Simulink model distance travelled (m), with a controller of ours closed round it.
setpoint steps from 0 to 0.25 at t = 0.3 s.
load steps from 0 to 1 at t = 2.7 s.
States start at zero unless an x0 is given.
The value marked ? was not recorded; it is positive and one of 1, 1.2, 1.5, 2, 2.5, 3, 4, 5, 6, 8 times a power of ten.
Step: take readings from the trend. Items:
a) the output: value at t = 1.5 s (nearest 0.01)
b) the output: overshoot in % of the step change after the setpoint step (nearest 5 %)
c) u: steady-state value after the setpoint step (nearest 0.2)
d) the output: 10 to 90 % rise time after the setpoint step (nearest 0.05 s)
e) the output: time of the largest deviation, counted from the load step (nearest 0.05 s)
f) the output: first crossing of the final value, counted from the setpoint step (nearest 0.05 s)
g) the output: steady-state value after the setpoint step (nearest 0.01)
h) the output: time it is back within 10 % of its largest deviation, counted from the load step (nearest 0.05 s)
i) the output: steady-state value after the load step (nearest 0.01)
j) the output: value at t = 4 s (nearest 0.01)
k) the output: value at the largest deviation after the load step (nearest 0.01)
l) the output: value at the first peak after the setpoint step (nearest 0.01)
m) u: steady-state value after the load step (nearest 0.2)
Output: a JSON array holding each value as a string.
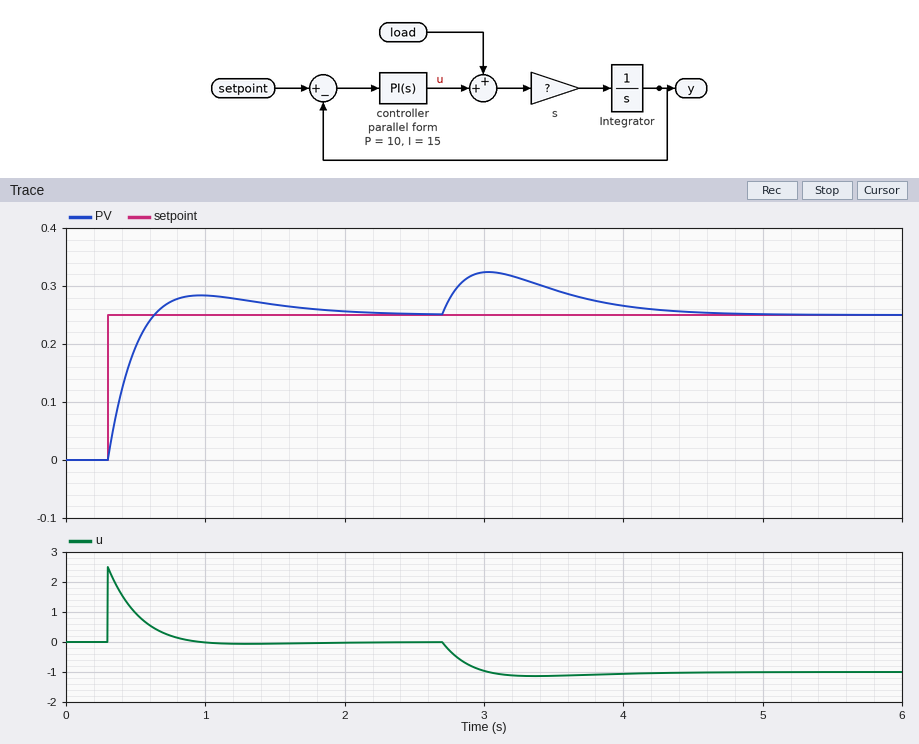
["0.27", "15 %", "0.0", "0.25 s", "0.35 s", "0.35 s", "0.25", "1.65 s", "0.25", "0.27", "0.32", "0.28", "-1.0"]
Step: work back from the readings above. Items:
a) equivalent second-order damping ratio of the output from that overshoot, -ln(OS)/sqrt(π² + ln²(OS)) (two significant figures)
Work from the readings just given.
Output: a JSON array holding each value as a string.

["0.52"]
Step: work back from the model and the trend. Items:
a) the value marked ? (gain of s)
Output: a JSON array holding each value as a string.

["0.6"]
